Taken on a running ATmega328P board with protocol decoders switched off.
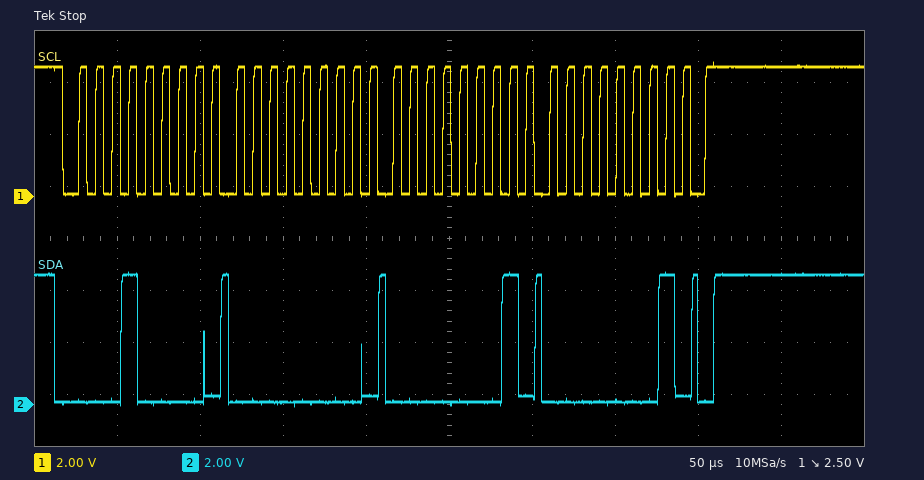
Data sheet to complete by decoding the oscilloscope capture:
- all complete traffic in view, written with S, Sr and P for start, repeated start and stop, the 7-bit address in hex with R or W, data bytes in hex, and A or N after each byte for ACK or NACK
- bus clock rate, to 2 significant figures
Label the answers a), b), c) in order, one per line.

a) S 08W A 00 A 01 A 01 A P
b) 100 kHz
